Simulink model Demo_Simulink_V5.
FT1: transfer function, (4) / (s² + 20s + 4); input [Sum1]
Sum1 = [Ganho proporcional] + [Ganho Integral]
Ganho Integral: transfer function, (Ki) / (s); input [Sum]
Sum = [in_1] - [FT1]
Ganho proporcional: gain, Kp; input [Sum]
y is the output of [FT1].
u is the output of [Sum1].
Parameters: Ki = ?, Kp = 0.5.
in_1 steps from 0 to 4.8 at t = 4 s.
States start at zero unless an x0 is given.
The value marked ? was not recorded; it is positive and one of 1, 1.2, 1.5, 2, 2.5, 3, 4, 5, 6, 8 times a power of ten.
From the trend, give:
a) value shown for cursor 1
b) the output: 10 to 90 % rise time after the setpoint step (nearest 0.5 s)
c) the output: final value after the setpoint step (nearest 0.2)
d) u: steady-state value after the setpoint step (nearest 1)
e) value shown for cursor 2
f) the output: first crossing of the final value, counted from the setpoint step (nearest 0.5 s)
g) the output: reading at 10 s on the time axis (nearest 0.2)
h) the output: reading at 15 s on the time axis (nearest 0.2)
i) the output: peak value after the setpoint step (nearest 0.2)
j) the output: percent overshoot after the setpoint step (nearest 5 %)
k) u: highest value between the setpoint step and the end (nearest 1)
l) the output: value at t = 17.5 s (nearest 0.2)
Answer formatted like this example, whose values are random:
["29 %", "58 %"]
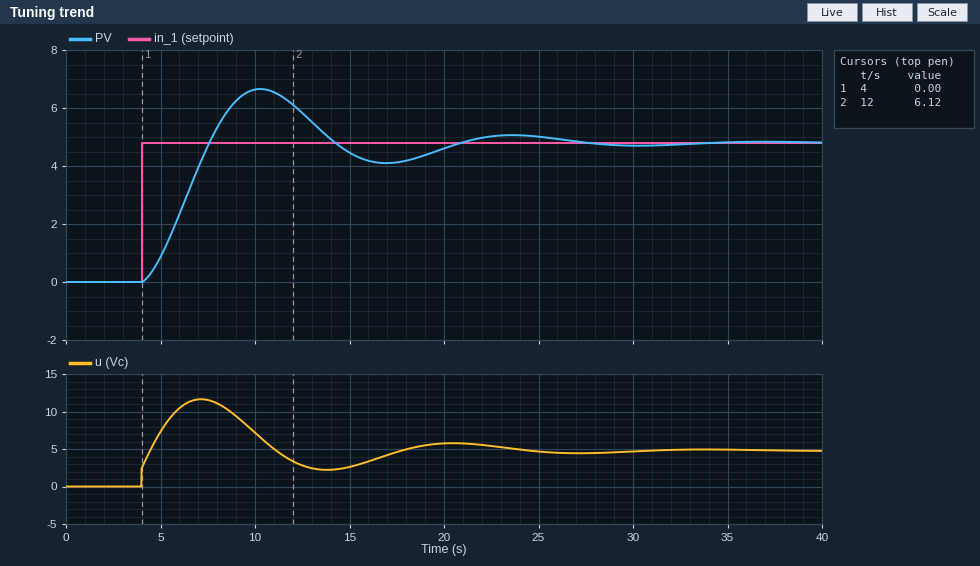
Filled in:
["0.00", "2.5 s", "4.8", "5", "6.12", "3.5 s", "6.6", "4.4", "6.6", "40 %", "12", "4.2"]
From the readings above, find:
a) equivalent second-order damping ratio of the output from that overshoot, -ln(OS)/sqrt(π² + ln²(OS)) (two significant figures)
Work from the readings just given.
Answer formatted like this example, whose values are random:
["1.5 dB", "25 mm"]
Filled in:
["0.28"]
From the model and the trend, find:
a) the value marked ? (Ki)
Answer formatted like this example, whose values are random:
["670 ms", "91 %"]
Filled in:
["1.2"]
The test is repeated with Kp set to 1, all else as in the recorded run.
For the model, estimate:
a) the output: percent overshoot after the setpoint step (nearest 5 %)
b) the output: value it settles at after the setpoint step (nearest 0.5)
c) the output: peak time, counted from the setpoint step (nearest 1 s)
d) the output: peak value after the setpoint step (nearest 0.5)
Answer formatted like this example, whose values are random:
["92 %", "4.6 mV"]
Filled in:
["30 %", "5.0", "6 s", "6.0"]
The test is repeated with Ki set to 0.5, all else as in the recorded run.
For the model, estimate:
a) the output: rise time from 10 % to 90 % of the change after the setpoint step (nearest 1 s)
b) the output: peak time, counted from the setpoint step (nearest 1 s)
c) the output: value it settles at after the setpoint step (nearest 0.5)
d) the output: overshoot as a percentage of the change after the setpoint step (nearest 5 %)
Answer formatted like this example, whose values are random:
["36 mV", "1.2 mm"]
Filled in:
["5 s", "10 s", "5.0", "20 %"]
